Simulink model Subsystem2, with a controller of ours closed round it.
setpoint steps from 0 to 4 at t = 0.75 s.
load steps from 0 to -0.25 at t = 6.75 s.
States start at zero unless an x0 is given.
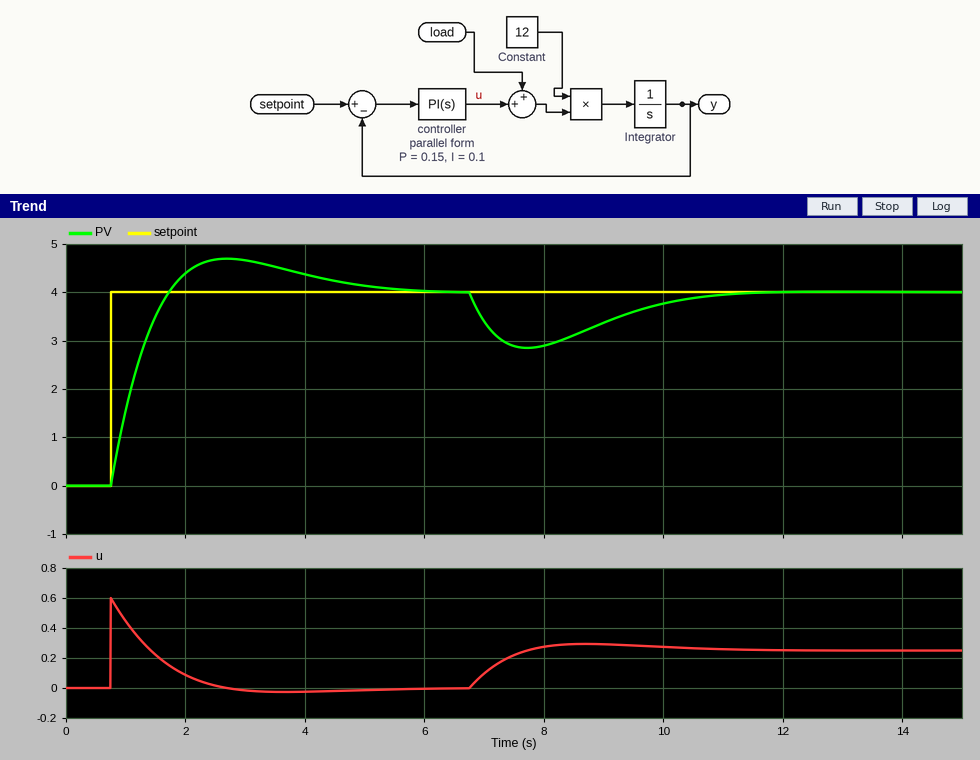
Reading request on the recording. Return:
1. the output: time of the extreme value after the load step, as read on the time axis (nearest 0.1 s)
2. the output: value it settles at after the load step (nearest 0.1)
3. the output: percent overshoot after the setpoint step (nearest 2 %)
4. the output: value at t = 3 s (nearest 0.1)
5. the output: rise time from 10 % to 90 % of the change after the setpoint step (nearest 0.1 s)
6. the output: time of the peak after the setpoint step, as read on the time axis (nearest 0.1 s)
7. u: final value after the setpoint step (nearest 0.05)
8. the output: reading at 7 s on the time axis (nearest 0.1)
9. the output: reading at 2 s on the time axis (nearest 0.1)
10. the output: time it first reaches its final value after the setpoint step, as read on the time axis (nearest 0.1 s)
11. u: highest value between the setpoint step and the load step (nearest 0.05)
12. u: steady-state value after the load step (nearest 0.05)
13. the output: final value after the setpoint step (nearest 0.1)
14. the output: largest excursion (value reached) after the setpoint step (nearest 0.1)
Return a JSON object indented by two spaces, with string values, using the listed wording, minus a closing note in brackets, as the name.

{
  "the output: time of the extreme value after the load step, as read on the time axis": "7.7 s",
  "the output: value it settles at after the load step": "4.0",
  "the output: percent overshoot after the setpoint step": "18 %",
  "the output: value at t = 3 s": "4.7",
  "the output: rise time from 10 % to 90 % of the change after the setpoint step": "0.7 s",
  "the output: time of the peak after the setpoint step, as read on the time axis": "2.7 s",
  "u: final value after the setpoint step": "0.00",
  "the output: reading at 7 s on the time axis": "3.4",
  "the output: reading at 2 s on the time axis": "4.4",
  "the output: time it first reaches its final value after the setpoint step, as read on the time axis": "1.7 s",
  "u: highest value between the setpoint step and the load step": "0.60",
  "u: steady-state value after the load step": "0.25",
  "the output: final value after the setpoint step": "4.0",
  "the output: largest excursion (value reached) after the setpoint step": "4.7"
}
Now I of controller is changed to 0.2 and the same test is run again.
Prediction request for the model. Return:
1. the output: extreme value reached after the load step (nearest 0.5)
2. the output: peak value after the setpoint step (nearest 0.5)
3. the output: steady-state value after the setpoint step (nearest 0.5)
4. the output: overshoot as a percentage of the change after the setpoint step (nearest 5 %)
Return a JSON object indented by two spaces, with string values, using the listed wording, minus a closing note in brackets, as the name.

{
  "the output: extreme value reached after the load step": "3.0",
  "the output: peak value after the setpoint step": "5.0",
  "the output: steady-state value after the setpoint step": "4.0",
  "the output: overshoot as a percentage of the change after the setpoint step": "25 %"
}
